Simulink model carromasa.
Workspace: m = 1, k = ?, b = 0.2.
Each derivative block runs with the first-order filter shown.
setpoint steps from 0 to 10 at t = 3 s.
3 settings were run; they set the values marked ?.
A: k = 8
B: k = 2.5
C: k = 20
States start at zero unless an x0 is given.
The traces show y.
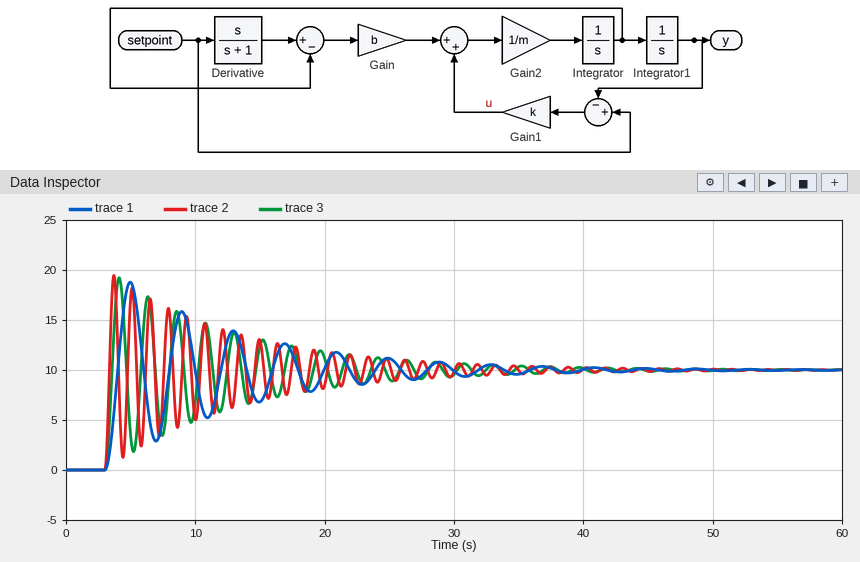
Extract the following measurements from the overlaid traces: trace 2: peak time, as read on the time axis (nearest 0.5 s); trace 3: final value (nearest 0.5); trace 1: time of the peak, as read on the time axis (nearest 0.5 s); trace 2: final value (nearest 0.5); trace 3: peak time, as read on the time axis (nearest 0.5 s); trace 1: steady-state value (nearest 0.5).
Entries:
3.5 s
10.0
5.0 s
10.0
4.0 s
10.0
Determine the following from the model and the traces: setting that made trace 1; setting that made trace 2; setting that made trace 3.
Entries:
B
C
A
